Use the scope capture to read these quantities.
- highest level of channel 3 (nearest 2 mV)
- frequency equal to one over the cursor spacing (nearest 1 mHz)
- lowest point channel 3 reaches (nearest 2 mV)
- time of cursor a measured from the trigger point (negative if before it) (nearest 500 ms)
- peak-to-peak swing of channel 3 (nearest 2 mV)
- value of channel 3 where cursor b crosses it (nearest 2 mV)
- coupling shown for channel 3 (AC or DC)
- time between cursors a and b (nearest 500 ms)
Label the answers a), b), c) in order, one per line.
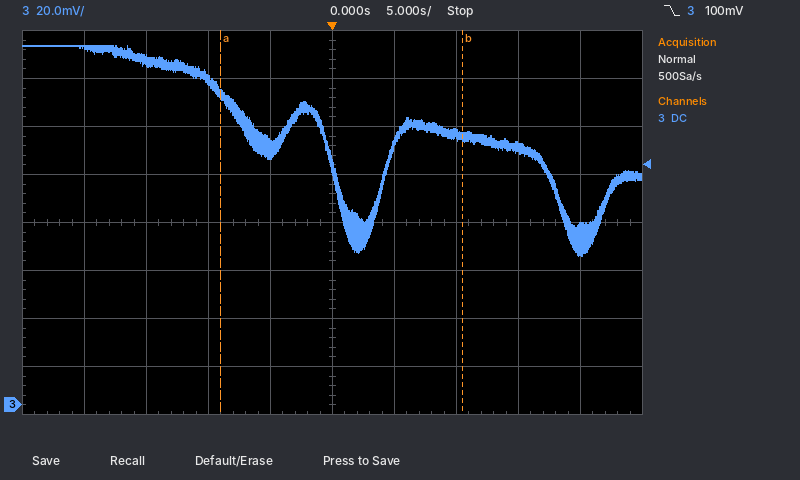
a) 150 mV
b) 51 mHz
c) 62 mV
d) -9.0 s
e) 88 mV
f) 112 mV
g) DC
h) 19.5 s
